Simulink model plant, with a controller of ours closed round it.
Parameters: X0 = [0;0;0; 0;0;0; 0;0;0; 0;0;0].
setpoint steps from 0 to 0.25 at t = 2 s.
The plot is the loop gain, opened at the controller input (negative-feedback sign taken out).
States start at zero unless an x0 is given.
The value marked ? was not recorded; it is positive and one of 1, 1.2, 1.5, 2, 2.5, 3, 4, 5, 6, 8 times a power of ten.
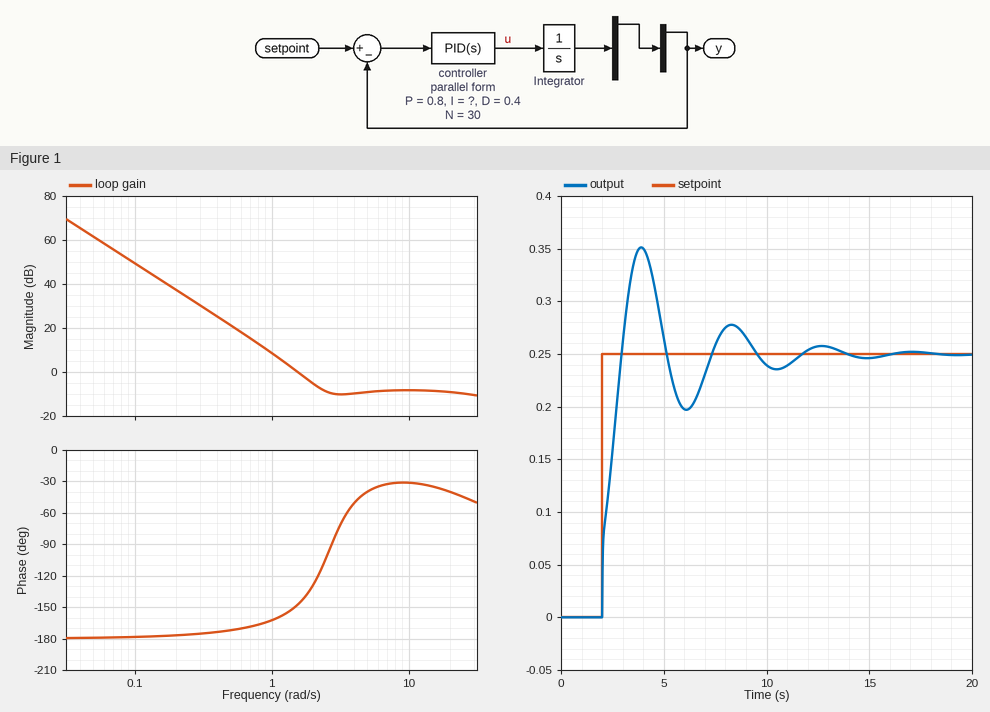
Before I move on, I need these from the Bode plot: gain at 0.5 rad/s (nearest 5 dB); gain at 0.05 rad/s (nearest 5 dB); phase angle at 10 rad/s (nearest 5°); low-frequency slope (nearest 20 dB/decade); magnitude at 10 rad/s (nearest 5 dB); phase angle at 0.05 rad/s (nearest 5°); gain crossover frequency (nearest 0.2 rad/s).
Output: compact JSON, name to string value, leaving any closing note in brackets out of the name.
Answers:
{"gain at 0.5 rad/s": "20 dB", "gain at 0.05 rad/s": "60 dB", "phase angle at 10 rad/s": "-30°", "low-frequency slope": "-40 dB/decade", "magnitude at 10 rad/s": "-10 dB", "phase angle at 0.05 rad/s": "-180°", "gain crossover frequency": "1.6 rad/s"}
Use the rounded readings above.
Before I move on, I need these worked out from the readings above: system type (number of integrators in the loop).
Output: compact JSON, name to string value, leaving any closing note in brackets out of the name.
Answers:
{"system type": "2"}
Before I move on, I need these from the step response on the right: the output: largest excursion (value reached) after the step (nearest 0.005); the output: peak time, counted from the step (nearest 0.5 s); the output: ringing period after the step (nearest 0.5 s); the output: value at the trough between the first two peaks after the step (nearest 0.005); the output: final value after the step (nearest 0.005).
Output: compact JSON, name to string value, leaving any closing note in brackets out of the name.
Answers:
{"the output: largest excursion (value reached) after the step": "0.350", "the output: peak time, counted from the step": "2.0 s", "the output: ringing period after the step": "4.5 s", "the output: value at the trough between the first two peaks after the step": "0.195", "the output: final value after the step": "0.250"}
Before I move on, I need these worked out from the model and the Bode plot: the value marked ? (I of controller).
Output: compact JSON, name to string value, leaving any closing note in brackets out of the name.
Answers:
{"the value marked ?": "3"}
